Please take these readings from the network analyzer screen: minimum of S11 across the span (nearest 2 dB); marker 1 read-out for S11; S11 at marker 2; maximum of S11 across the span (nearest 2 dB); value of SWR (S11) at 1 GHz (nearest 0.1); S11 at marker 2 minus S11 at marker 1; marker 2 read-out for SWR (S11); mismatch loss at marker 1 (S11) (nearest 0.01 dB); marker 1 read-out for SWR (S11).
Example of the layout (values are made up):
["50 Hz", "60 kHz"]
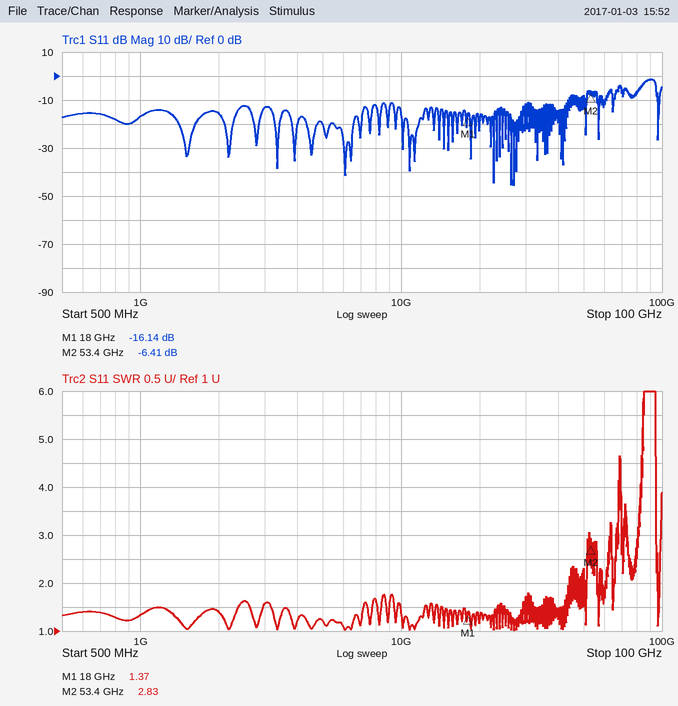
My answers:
["-46 dB", "-16.14 dB", "-6.41 dB", "-2 dB", "1.3", "9.73 dB", "2.83", "0.11 dB", "1.37"]
